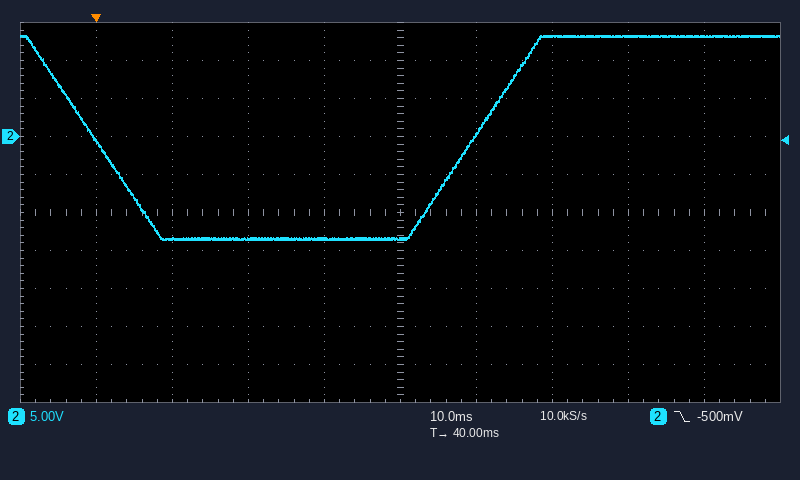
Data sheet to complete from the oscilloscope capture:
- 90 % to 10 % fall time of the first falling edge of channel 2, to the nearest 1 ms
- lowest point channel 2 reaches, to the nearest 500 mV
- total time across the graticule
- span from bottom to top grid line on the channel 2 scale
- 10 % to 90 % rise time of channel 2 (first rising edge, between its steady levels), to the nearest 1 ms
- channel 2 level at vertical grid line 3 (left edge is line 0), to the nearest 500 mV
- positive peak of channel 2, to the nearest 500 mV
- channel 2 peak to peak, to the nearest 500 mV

14 ms
-13.5 V
100 ms
50 V
14 ms
-13.5 V
13.5 V
27.0 V
